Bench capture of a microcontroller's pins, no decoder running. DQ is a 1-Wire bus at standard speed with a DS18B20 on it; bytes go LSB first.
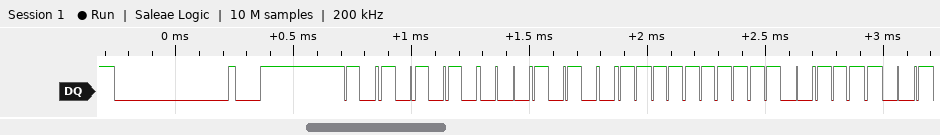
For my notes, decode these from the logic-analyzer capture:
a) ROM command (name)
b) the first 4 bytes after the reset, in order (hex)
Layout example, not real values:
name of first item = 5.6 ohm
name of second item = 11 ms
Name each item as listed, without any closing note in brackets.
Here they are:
ROM command = Match ROM
the first 4 bytes after the reset, in order = 55 28 FF F3
